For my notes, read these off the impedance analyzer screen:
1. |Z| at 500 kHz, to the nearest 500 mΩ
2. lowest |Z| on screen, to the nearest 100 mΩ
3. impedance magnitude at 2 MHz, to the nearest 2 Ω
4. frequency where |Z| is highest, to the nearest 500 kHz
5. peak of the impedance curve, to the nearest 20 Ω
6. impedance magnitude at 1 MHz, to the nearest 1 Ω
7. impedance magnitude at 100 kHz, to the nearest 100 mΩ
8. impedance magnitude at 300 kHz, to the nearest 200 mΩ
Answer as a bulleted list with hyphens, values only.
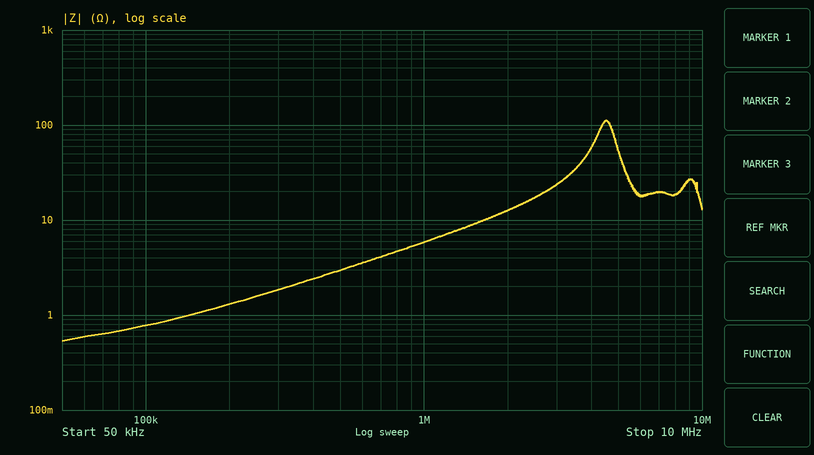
- 3.0 Ω
- 500 mΩ
- 12 Ω
- 4.5 MHz
- 120 Ω
- 6 Ω
- 800 mΩ
- 1.8 Ω
